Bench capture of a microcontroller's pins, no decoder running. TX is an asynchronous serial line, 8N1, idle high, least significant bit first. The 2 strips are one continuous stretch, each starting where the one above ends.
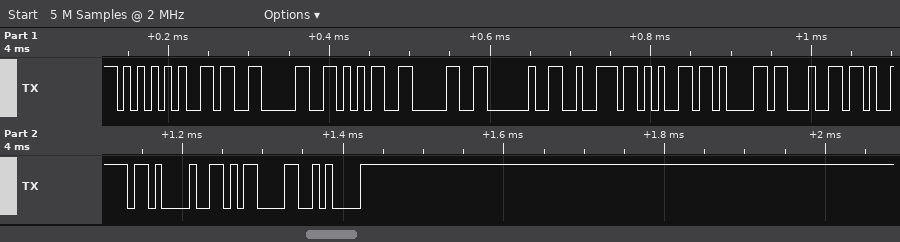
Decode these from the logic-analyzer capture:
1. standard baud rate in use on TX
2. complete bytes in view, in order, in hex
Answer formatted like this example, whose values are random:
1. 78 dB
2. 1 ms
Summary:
1. 115200 baud
2. 55 36 30 35 30 20 72 65 61 64 79 21 0D 0A
